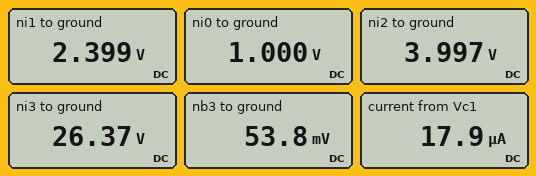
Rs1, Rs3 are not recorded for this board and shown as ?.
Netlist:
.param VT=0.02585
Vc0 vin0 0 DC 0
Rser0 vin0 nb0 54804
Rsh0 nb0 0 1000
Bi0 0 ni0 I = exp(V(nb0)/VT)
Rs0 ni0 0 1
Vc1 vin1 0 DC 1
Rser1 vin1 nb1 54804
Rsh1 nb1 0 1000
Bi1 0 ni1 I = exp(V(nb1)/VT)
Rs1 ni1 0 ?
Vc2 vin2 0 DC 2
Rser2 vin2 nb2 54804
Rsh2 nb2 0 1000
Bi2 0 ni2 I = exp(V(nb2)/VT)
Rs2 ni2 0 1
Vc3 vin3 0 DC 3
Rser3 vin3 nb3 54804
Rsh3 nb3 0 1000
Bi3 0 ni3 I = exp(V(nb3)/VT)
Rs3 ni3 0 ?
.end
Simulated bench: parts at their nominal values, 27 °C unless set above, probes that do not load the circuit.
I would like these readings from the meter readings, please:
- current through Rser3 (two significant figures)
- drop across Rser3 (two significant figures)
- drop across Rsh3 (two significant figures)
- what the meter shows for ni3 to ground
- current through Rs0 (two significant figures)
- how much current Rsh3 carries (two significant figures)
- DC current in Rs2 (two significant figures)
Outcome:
54 µA
2.9 V
54 mV
26.37 V
1.0 A
54 µA
4.0 A
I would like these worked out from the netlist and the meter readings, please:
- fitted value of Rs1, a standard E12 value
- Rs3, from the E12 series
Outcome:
1.2 Ω
3.3 Ω
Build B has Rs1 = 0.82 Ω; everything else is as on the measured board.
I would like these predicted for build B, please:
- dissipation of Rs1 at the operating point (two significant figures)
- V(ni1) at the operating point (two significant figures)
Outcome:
3.3 W
1.6 V
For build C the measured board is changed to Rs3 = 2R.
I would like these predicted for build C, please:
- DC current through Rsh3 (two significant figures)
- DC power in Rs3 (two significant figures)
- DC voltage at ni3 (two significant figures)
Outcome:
54 µA
130 W
16 V
